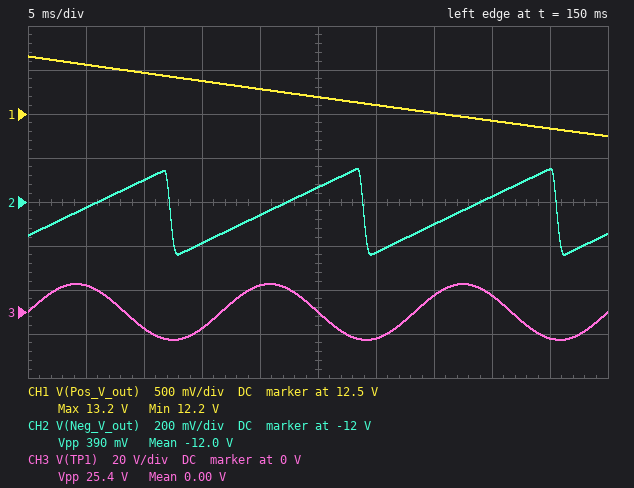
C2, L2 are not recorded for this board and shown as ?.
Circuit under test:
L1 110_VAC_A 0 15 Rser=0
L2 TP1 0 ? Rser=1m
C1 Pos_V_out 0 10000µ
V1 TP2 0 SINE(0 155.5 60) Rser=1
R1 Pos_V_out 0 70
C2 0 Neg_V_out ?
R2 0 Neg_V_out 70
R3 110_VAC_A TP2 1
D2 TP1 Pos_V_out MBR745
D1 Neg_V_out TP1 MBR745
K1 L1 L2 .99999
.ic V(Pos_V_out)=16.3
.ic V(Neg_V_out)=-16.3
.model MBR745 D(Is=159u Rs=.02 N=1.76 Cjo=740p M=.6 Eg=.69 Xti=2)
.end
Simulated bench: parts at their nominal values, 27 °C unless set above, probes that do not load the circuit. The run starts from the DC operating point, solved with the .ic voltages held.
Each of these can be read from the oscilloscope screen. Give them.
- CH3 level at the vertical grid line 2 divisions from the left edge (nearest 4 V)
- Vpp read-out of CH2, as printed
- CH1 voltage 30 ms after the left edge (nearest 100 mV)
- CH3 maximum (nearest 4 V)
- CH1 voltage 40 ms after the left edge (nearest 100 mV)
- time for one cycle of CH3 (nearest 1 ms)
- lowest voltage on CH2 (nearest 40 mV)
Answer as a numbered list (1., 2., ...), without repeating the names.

1. -8 V
2. 390 mV
3. 12.6 V
4. 12 V
5. 12.4 V
6. 17 ms
7. -12.24 V
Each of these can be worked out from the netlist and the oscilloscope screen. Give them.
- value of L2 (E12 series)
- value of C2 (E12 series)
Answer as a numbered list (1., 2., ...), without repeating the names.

1. 100 mH
2. 6.8 mF
